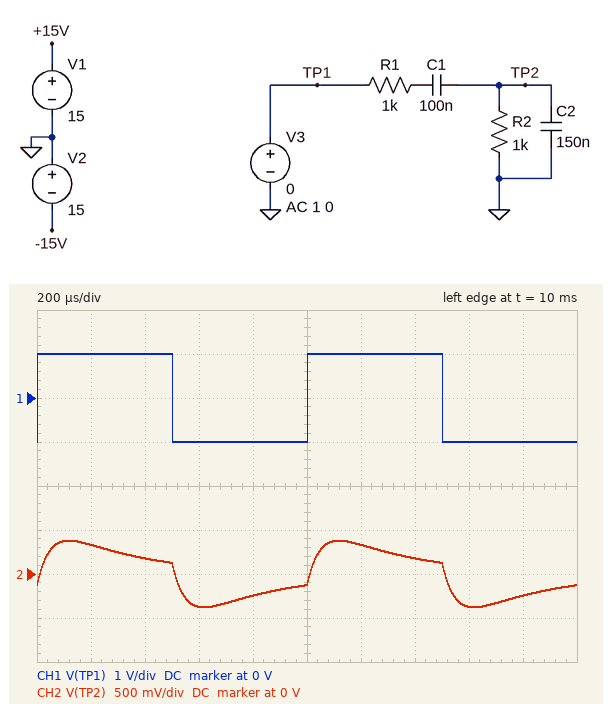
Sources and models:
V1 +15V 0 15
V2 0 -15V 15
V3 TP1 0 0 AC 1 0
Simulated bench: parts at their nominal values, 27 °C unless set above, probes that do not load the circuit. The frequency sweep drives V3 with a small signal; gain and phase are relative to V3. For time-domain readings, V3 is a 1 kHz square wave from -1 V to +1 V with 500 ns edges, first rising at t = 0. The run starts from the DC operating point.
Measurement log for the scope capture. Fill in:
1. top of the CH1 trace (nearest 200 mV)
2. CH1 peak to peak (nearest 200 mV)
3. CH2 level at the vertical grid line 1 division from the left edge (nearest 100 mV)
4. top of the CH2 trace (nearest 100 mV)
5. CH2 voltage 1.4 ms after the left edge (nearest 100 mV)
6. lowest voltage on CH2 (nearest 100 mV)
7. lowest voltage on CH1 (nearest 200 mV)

1.0 V
2.0 V
300 mV
400 mV
200 mV
-400 mV
-1.0 V
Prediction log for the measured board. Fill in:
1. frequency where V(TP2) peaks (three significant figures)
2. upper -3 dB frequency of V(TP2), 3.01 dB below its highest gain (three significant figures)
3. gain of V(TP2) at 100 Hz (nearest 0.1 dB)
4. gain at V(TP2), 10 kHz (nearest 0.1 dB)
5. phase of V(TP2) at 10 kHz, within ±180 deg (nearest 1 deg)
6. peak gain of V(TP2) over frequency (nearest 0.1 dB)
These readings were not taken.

1.30 kHz
4.12 kHz
-24.2 dB
-19.9 dB
-69 deg
-10.9 dB
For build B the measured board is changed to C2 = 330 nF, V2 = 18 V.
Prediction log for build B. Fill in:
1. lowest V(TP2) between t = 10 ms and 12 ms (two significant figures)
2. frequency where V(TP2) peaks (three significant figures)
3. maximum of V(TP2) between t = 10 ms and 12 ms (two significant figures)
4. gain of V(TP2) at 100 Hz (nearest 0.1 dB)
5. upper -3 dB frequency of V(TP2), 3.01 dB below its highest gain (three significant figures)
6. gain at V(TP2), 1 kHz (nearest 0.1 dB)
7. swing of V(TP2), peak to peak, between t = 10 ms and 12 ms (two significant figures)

-220 mV
876 Hz
220 mV
-24.4 dB
2.83 kHz
-14.5 dB
440 mV
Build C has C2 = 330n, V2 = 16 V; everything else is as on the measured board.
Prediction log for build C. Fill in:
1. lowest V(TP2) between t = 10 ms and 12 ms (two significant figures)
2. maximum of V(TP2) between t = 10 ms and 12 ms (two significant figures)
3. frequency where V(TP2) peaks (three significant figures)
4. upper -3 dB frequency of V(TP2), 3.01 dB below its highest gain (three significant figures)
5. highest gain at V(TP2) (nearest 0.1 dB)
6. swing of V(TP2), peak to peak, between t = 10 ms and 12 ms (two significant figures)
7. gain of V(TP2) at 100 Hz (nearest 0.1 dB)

-220 mV
220 mV
876 Hz
2.83 kHz
-14.5 dB
440 mV
-24.4 dB
